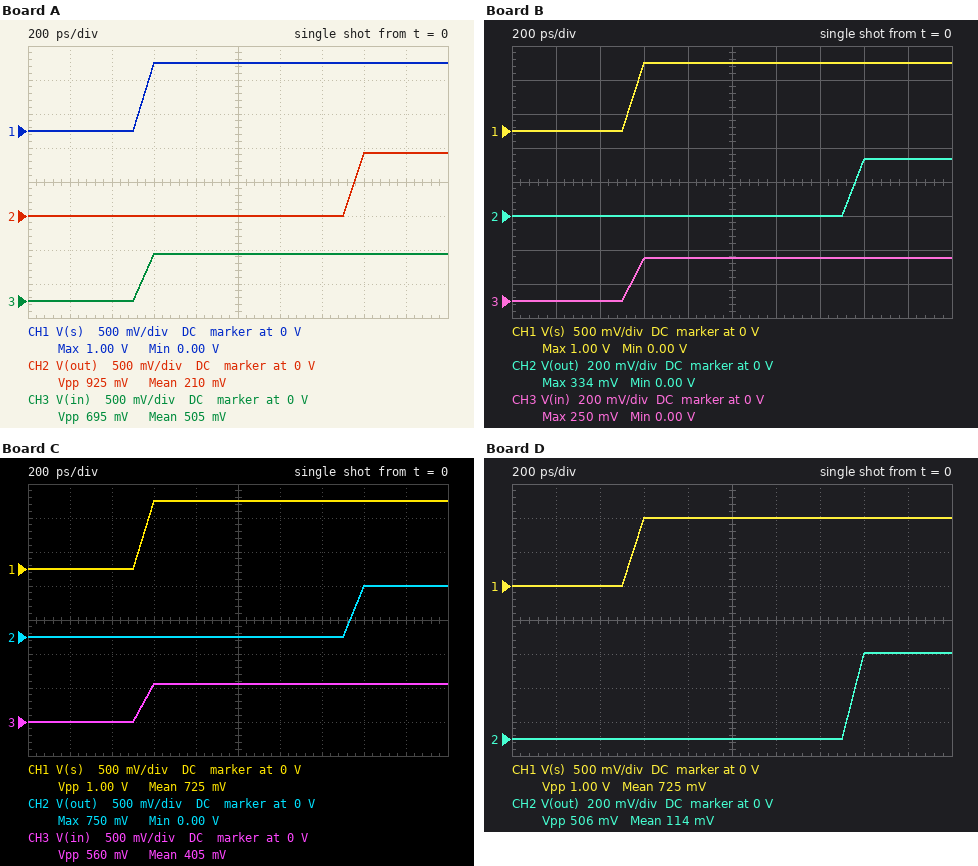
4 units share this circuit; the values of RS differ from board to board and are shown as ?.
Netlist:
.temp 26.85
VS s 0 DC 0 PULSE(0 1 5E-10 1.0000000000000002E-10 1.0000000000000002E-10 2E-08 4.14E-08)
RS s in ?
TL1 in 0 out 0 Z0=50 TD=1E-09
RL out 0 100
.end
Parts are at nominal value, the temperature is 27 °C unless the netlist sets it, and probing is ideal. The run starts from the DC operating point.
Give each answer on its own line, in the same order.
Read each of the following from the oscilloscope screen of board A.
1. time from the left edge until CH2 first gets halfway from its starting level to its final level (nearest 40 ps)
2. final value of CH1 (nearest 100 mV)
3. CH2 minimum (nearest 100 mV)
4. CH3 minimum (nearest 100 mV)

1.56 ns
1.0 V
0 V
0 V
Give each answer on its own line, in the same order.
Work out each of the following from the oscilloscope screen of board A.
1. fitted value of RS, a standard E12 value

22 Ω
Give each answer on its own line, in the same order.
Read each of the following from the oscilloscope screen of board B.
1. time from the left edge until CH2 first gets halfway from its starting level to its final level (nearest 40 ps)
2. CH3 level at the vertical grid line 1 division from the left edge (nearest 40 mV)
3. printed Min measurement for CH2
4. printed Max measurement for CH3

1.56 ns
0 V
0.00 V
250 mV
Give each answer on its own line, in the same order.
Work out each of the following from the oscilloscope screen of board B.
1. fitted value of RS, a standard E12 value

150 Ω
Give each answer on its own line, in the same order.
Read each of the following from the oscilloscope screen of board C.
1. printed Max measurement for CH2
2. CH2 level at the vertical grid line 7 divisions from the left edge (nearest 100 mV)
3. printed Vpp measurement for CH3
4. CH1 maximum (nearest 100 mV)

750 mV
0 V
560 mV
1.0 V
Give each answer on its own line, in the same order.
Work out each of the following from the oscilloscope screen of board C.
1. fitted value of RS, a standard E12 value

39 Ω
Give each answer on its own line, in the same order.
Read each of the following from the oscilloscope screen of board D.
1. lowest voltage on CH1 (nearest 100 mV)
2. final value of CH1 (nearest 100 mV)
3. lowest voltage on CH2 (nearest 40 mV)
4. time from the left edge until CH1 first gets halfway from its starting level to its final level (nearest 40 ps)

0 V
1.0 V
0 V
560 ps
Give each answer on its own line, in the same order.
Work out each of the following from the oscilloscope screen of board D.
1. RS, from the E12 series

82 Ω
